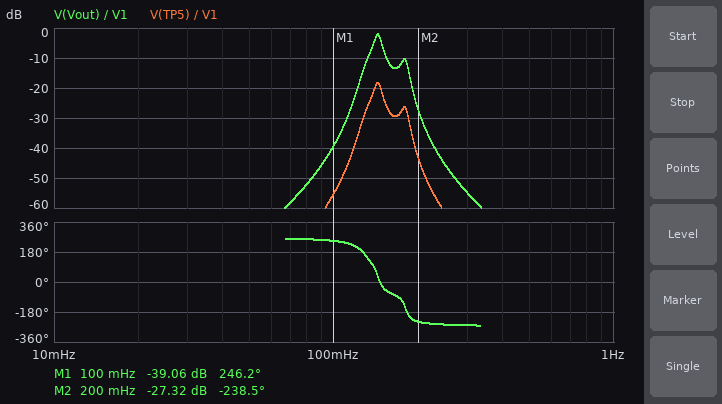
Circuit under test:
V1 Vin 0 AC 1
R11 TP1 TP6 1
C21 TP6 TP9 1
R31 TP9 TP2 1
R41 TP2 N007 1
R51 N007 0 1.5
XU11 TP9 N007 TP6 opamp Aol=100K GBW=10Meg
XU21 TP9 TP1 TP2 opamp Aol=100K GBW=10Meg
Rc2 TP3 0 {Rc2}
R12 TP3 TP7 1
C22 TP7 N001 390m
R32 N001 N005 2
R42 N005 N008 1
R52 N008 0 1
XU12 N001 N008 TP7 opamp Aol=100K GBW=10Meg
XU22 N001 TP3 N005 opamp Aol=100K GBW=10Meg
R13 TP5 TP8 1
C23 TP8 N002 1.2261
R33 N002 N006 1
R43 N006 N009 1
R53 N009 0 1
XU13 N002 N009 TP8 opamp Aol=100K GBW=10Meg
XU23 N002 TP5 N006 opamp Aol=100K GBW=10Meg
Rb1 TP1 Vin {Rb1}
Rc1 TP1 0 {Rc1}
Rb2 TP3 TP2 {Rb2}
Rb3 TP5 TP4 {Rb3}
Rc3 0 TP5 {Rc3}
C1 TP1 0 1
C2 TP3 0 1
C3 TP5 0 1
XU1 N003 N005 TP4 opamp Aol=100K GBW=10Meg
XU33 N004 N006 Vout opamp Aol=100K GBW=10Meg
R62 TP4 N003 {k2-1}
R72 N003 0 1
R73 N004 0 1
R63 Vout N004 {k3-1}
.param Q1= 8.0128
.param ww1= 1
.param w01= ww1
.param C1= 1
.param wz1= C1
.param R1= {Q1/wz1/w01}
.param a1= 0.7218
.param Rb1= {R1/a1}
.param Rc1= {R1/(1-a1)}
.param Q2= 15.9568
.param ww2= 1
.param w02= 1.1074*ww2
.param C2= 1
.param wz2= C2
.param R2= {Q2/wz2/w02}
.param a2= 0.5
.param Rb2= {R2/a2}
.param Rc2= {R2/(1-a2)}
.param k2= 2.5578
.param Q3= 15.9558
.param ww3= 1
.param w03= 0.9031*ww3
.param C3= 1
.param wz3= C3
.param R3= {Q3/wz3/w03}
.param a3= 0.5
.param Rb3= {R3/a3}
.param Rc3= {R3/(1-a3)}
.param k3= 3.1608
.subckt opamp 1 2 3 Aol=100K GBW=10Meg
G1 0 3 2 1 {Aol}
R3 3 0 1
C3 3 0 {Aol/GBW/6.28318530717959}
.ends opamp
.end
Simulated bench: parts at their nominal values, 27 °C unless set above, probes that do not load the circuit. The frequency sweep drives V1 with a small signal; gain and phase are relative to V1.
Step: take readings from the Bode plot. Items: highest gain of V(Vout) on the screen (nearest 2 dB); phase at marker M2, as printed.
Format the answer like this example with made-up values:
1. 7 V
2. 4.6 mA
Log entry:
1. -2 dB
2. -238.5 deg
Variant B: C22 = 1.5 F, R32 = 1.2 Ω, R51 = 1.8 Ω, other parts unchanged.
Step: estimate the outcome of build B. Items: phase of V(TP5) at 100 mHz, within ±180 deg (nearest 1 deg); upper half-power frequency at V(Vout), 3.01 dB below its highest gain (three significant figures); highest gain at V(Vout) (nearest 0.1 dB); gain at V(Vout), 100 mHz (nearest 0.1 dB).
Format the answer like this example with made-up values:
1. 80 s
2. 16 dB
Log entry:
1. -136 deg
2. 126 mHz
3. 3.4 dB
4. -21.1 dB
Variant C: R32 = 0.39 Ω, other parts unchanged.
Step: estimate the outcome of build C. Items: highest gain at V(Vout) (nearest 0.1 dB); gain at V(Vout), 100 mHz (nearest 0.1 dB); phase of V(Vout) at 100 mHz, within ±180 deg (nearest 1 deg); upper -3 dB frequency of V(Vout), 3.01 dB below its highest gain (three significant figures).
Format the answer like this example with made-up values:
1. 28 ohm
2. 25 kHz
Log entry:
1. -23.8 dB
2. -55.9 dB
3. -111 deg
4. 147 mHz
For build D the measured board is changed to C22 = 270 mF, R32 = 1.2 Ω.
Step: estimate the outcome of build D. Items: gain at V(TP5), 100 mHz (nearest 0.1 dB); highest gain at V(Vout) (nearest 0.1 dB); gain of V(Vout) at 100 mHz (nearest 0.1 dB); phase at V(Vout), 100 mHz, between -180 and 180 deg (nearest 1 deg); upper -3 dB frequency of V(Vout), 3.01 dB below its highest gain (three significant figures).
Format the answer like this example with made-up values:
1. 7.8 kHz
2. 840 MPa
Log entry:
1. -64.7 dB
2. -15.7 dB
3. -48.7 dB
4. -112 deg
5. 147 mHz
